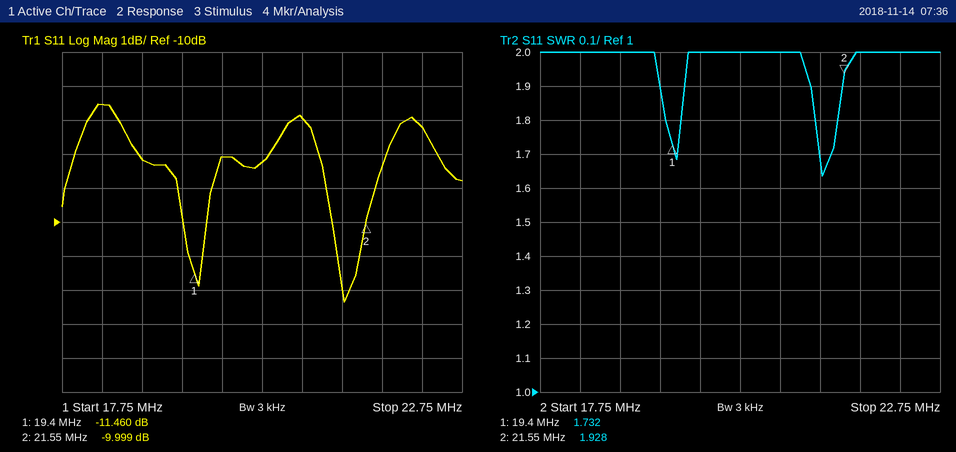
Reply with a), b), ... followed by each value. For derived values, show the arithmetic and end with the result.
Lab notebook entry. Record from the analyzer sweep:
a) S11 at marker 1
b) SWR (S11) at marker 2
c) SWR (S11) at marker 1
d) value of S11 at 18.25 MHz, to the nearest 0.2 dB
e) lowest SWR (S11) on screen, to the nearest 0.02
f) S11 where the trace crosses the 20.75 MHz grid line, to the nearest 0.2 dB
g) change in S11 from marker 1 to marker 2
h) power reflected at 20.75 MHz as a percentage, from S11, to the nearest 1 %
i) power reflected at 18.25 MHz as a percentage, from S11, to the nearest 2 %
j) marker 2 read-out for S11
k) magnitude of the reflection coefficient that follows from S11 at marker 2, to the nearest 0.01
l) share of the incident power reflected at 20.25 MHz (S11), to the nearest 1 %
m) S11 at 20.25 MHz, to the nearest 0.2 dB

a) -11.460 dB
b) 1.928
c) 1.732
d) -6.6 dB
e) 1.64
f) -7.0 dB
g) -9.999 − (-11.46) = 1.461 dB
h) 10^(-7/10) ≈ 20 %
i) 10^(-6.6/10) ≈ 22 %
j) -9.999 dB
k) 10^(-9.999/20) ≈ 0.32
l) 10^(-8.2/10) ≈ 15 %
m) -8.2 dB
